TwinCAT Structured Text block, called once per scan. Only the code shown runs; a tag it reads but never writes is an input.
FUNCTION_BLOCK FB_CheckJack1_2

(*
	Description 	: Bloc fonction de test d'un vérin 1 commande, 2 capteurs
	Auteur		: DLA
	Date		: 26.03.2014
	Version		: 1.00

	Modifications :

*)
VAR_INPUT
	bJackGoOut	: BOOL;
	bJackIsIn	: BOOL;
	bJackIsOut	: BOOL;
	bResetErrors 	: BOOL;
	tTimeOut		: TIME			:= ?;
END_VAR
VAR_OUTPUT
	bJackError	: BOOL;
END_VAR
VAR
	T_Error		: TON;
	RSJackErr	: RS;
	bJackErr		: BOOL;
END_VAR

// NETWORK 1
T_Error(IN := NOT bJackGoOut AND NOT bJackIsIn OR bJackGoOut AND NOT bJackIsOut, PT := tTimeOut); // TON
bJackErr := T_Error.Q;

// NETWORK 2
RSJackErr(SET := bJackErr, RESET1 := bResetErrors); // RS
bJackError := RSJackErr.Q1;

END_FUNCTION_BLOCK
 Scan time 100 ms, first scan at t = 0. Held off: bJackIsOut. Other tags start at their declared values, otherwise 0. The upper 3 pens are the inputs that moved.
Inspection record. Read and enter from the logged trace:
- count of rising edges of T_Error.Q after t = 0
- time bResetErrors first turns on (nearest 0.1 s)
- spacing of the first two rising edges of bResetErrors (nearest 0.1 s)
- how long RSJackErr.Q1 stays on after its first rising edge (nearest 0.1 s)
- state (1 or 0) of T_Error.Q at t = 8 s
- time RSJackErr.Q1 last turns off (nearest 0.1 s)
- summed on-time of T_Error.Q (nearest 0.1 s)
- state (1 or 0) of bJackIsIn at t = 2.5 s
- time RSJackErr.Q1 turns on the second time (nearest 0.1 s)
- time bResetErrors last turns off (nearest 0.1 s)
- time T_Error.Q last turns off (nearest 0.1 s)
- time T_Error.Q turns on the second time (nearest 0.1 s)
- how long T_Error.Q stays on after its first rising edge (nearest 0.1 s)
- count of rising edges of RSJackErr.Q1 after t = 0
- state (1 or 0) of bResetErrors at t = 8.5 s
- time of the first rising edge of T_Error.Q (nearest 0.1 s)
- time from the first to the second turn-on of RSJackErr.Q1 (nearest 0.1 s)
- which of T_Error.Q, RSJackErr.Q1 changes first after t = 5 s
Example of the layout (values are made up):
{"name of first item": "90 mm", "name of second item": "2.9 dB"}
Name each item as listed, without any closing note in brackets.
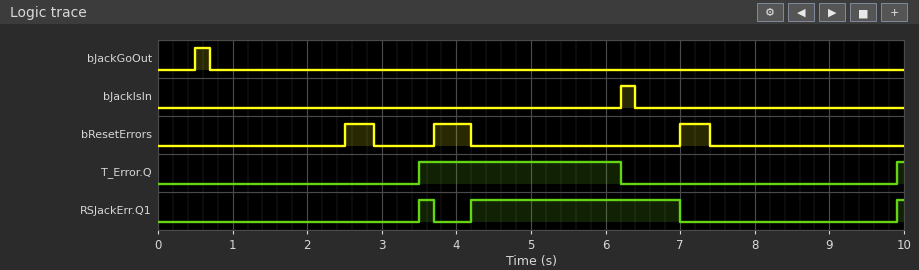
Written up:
{"count of rising edges of T_Error.Q after t = 0": "2", "time bResetErrors first turns on": "2.5 s", "spacing of the first two rising edges of bResetErrors": "1.2 s", "how long RSJackErr.Q1 stays on after its first rising edge": "0.2 s", "state (1 or 0) of T_Error.Q at t = 8 s": "0", "time RSJackErr.Q1 last turns off": "7.0 s", "summed on-time of T_Error.Q": "2.8 s", "state (1 or 0) of bJackIsIn at t = 2.5 s": "0", "time RSJackErr.Q1 turns on the second time": "4.2 s", "time bResetErrors last turns off": "7.4 s", "time T_Error.Q last turns off": "6.2 s", "time T_Error.Q turns on the second time": "9.9 s", "how long T_Error.Q stays on after its first rising edge": "2.7 s", "count of rising edges of RSJackErr.Q1 after t = 0": "3", "state (1 or 0) of bResetErrors at t = 8.5 s": "0", "time of the first rising edge of T_Error.Q": "3.5 s", "time from the first to the second turn-on of RSJackErr.Q1": "0.7 s", "which of T_Error.Q, RSJackErr.Q1 changes first after t = 5 s": "T_Error.Q"}
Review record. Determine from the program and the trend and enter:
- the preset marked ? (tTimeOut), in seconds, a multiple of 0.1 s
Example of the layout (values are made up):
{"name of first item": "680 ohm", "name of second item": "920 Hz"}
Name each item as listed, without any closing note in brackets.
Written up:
{"the preset marked ? (tTimeOut), in seconds, a multiple of 0.1 s": "3.5 s"}
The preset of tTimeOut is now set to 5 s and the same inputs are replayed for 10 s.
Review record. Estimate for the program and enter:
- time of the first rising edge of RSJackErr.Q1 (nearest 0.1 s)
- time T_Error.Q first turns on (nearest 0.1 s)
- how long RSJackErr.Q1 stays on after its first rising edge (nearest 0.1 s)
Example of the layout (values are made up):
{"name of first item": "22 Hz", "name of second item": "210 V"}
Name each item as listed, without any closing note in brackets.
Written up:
{"time of the first rising edge of RSJackErr.Q1": "5.0 s", "time T_Error.Q first turns on": "5.0 s", "how long RSJackErr.Q1 stays on after its first rising edge": "2.0 s"}
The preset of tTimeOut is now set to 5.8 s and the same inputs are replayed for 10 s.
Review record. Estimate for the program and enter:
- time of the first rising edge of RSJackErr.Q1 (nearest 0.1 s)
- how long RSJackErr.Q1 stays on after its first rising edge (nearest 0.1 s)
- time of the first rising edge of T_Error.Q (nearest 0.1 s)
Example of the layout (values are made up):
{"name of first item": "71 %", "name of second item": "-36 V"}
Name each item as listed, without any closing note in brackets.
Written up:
{"time of the first rising edge of RSJackErr.Q1": "5.8 s", "how long RSJackErr.Q1 stays on after its first rising edge": "1.2 s", "time of the first rising edge of T_Error.Q": "5.8 s"}
